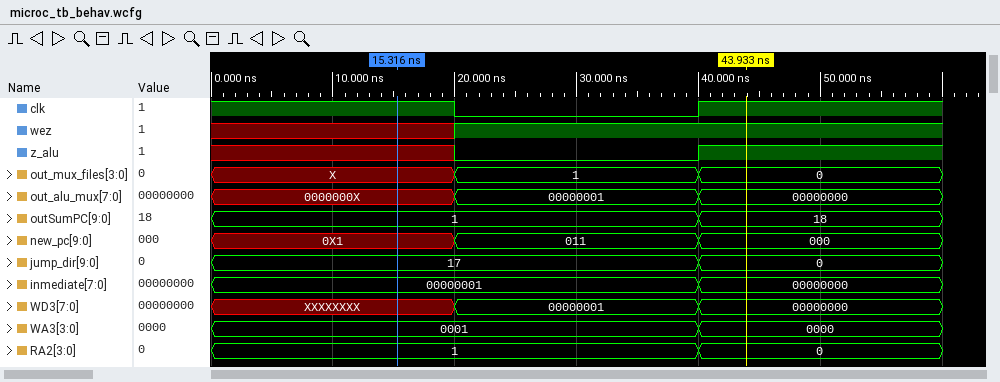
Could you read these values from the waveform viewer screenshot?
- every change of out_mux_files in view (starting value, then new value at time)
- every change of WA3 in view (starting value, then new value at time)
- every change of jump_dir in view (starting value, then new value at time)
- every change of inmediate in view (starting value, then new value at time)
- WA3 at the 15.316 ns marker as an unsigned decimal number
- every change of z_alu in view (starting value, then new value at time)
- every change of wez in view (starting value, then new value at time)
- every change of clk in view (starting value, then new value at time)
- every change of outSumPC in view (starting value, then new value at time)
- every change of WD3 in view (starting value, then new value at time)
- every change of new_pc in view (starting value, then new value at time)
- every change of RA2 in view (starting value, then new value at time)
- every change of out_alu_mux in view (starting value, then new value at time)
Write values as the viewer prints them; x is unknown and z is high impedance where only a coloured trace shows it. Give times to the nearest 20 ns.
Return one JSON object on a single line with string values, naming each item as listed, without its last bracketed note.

{"every change of out_mux_files in view": "X, 1 at 20 ns, 0 at 40 ns", "every change of WA3 in view": "0001, 0000 at 40 ns", "every change of jump_dir in view": "17, 0 at 40 ns", "every change of inmediate in view": "00000001, 00000000 at 40 ns", "WA3 at the 15.316 ns marker as an unsigned decimal number": "1", "every change of z_alu in view": "x, 0 at 20 ns, 1 at 40 ns", "every change of wez in view": "x, 1 at 20 ns", "every change of clk in view": "1, 0 at 20 ns, 1 at 40 ns", "every change of outSumPC in view": "1, 18 at 40 ns", "every change of WD3 in view": "XXXXXXXX, 00000001 at 20 ns, 00000000 at 40 ns", "every change of new_pc in view": "0X1, 011 at 20 ns, 000 at 40 ns", "every change of RA2 in view": "1, 0 at 40 ns", "every change of out_alu_mux in view": "0000000X, 00000001 at 20 ns, 00000000 at 40 ns"}
